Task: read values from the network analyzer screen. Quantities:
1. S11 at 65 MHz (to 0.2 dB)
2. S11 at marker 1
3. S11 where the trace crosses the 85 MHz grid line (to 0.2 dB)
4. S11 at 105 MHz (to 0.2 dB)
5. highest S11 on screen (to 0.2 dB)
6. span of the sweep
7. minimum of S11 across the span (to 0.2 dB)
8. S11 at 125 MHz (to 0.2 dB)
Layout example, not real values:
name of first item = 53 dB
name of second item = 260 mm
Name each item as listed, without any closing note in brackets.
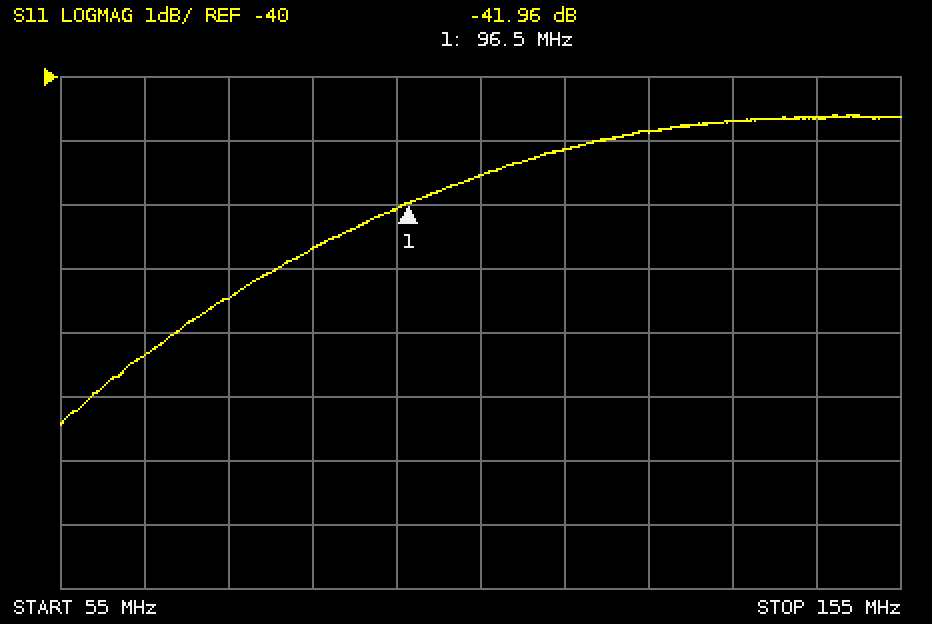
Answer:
S11 at 65 MHz = -44.4 dB
S11 at marker 1 = -41.96 dB
S11 where the trace crosses the 85 MHz grid line = -42.6 dB
S11 at 105 MHz = -41.6 dB
highest S11 on screen = -40.6 dB
span of the sweep = 100 MHz
minimum of S11 across the span = -45.4 dB
S11 at 125 MHz = -40.8 dB
